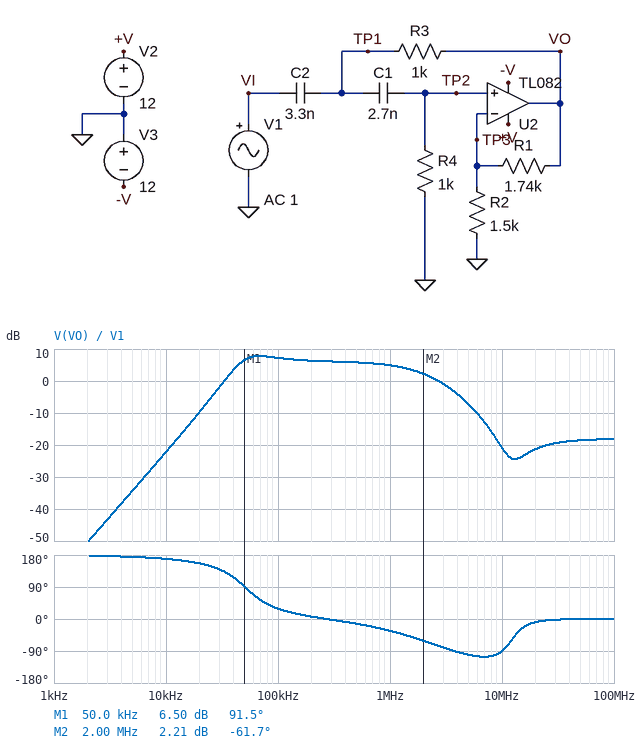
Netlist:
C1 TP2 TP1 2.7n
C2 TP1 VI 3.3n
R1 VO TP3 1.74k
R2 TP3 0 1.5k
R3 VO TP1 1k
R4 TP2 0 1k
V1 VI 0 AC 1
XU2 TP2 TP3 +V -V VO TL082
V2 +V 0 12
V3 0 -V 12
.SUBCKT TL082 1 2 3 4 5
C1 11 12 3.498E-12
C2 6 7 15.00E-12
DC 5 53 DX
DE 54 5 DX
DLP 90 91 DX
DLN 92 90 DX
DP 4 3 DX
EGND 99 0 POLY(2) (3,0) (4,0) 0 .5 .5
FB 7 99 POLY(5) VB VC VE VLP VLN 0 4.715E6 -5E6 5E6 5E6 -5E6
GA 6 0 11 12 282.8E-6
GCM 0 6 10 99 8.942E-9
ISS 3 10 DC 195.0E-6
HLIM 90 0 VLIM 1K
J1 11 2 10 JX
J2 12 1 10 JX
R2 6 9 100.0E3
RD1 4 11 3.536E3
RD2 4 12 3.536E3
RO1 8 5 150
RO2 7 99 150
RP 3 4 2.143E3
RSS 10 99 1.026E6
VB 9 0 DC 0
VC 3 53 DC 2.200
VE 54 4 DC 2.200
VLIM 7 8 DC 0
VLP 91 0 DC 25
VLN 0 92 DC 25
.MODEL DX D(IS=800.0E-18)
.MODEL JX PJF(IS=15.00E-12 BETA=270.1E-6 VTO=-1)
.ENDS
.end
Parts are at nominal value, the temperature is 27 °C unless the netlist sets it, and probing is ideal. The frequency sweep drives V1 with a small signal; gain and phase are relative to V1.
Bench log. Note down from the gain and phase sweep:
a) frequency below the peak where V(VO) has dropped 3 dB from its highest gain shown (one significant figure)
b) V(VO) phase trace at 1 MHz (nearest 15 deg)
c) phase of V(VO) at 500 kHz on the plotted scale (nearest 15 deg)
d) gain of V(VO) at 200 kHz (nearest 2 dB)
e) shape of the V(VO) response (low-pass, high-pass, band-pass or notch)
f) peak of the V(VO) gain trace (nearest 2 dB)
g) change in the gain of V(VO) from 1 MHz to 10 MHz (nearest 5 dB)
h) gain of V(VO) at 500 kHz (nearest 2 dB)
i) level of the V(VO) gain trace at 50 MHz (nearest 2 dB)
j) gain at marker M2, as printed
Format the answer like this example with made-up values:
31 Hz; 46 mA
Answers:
40 kHz; -30 deg; -15 deg; 6 dB; band-pass; 8 dB; -25 dB; 6 dB; -18 dB; 2.21 dB
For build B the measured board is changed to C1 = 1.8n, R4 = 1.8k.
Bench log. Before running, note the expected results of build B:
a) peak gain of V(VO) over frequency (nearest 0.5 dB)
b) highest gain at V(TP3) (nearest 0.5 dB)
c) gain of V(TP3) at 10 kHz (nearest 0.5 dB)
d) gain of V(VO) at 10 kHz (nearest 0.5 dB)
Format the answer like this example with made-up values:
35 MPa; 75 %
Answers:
14.5 dB; 7.5 dB; -27.0 dB; -20.5 dB
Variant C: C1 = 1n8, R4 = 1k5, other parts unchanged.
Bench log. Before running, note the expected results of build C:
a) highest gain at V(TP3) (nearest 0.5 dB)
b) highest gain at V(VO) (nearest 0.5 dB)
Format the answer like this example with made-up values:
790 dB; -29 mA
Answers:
4.0 dB; 10.5 dB
